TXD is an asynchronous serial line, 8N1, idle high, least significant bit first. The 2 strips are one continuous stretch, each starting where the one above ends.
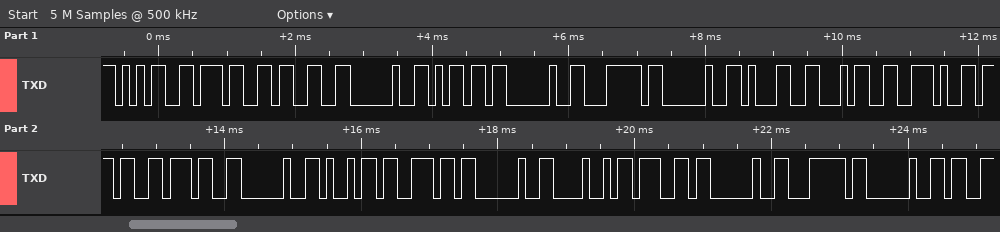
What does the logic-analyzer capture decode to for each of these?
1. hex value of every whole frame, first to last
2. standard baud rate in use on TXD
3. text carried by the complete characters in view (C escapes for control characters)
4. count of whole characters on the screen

35 37 33 20 6D 20 7C 20 31 34 2E 37 37 20 69 6E 20 48 67 20 7C 20
9600 baud
"573 m | 14.77 in Hg | "
22
